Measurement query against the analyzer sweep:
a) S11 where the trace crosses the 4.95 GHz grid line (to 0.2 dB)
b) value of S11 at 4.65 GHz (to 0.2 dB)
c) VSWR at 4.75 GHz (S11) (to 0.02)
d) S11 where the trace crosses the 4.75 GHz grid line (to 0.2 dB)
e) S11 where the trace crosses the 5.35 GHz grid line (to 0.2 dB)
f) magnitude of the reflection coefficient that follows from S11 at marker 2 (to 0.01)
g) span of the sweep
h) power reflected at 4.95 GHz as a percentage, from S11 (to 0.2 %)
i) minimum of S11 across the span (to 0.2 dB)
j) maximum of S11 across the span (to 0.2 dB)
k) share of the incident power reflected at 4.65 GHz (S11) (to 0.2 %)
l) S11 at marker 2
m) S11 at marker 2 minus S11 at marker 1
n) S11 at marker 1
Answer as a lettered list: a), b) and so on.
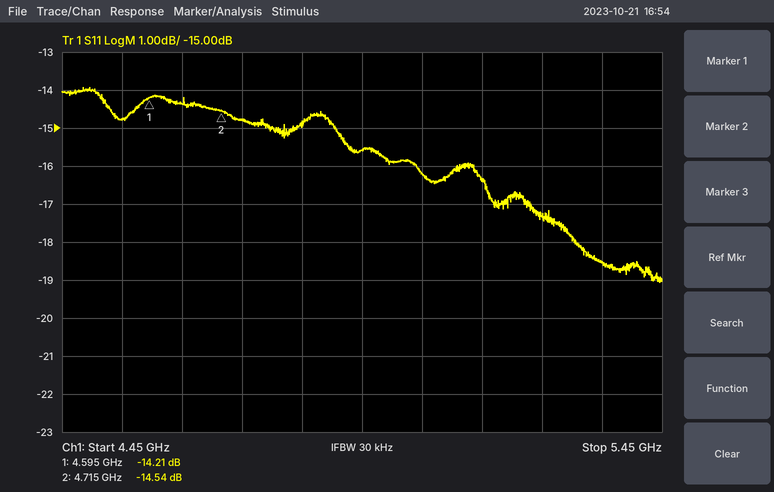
a) -15.6 dB
b) -14.4 dB
c) 1.44
d) -14.8 dB
e) -18.6 dB
f) 0.19
g) 1 GHz
h) 2.8 %
i) -19.0 dB
j) -14.0 dB
k) 3.6 %
l) -14.54 dB
m) -0.33 dB
n) -14.21 dB
